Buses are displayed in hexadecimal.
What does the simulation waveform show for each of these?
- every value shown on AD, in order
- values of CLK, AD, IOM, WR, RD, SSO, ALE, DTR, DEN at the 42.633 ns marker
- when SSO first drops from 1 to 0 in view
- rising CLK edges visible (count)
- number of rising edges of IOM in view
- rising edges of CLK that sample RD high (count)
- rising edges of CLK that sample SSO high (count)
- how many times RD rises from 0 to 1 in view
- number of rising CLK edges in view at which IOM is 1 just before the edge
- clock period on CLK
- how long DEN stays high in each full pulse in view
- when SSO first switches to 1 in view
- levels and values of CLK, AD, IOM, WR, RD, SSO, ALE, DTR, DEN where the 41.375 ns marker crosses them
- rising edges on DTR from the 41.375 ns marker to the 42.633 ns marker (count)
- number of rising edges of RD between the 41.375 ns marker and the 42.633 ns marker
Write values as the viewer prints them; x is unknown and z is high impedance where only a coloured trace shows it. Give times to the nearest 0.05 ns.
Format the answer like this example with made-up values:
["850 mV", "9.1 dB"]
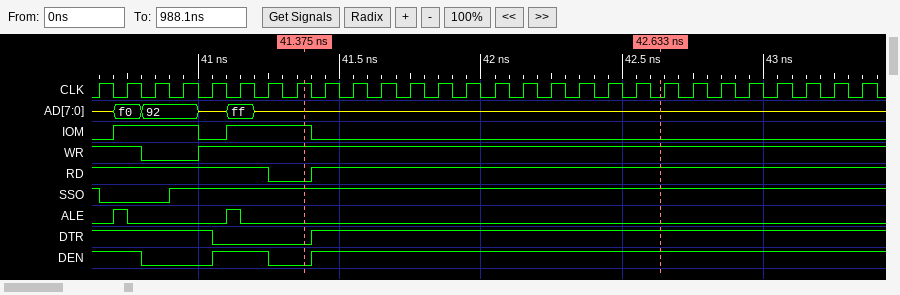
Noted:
["z, f0, 92, z, ff, z", "CLK=0, AD=z, IOM=0, WR=1, RD=1, SSO=1, ALE=0, DTR=1, DEN=1", "40.65 ns", "28", "2", "27", "26", "1", "6", "0.1 ns", "0.2 ns", "40.9 ns", "CLK=1, AD=z, IOM=1, WR=1, RD=0, SSO=1, ALE=0, DTR=0, DEN=0", "1", "1"]
